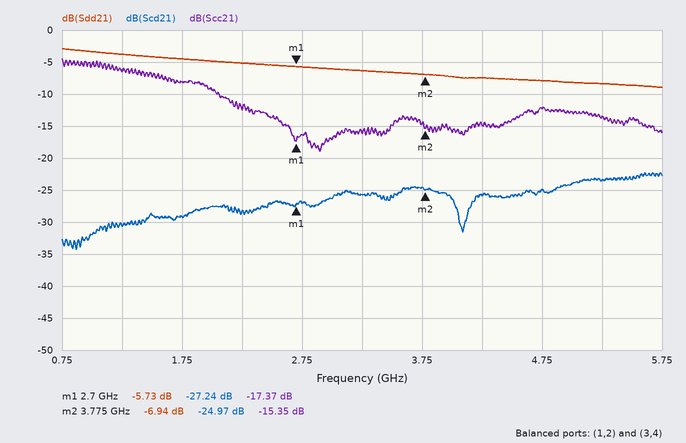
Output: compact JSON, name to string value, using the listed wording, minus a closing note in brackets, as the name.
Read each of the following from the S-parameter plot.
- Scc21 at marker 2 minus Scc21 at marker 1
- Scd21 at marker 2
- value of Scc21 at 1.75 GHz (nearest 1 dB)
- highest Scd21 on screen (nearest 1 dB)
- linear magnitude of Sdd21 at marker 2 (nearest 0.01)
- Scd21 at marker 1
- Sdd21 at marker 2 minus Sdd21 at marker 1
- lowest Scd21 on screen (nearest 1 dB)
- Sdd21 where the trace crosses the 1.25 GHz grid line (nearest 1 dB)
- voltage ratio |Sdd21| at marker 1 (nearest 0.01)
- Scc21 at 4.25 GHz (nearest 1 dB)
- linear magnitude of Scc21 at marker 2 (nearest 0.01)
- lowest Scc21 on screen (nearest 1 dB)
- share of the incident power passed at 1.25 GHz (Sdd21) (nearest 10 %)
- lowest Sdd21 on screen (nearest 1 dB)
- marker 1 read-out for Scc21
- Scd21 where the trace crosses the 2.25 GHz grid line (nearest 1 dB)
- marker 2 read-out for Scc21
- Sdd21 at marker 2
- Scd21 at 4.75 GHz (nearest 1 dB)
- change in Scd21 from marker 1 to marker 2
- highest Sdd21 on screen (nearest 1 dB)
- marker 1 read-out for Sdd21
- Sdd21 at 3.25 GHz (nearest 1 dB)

{"Scc21 at marker 2 minus Scc21 at marker 1": "2.02 dB", "Scd21 at marker 2": "-24.97 dB", "value of Scc21 at 1.75 GHz": "-8 dB", "highest Scd21 on screen": "-22 dB", "linear magnitude of Sdd21 at marker 2": "0.45", "Scd21 at marker 1": "-27.24 dB", "Sdd21 at marker 2 minus Sdd21 at marker 1": "-1.21 dB", "lowest Scd21 on screen": "-34 dB", "Sdd21 where the trace crosses the 1.25 GHz grid line": "-4 dB", "voltage ratio |Sdd21| at marker 1": "0.52", "Scc21 at 4.25 GHz": "-15 dB", "linear magnitude of Scc21 at marker 2": "0.17", "lowest Scc21 on screen": "-19 dB", "share of the incident power passed at 1.25 GHz (Sdd21)": "40 %", "lowest Sdd21 on screen": "-9 dB", "marker 1 read-out for Scc21": "-17.37 dB", "Scd21 where the trace crosses the 2.25 GHz grid line": "-28 dB", "marker 2 read-out for Scc21": "-15.35 dB", "Sdd21 at marker 2": "-6.94 dB", "Scd21 at 4.75 GHz": "-25 dB", "change in Scd21 from marker 1 to marker 2": "2.27 dB", "highest Sdd21 on screen": "-3 dB", "marker 1 read-out for Sdd21": "-5.73 dB", "Sdd21 at 3.25 GHz": "-6 dB"}
